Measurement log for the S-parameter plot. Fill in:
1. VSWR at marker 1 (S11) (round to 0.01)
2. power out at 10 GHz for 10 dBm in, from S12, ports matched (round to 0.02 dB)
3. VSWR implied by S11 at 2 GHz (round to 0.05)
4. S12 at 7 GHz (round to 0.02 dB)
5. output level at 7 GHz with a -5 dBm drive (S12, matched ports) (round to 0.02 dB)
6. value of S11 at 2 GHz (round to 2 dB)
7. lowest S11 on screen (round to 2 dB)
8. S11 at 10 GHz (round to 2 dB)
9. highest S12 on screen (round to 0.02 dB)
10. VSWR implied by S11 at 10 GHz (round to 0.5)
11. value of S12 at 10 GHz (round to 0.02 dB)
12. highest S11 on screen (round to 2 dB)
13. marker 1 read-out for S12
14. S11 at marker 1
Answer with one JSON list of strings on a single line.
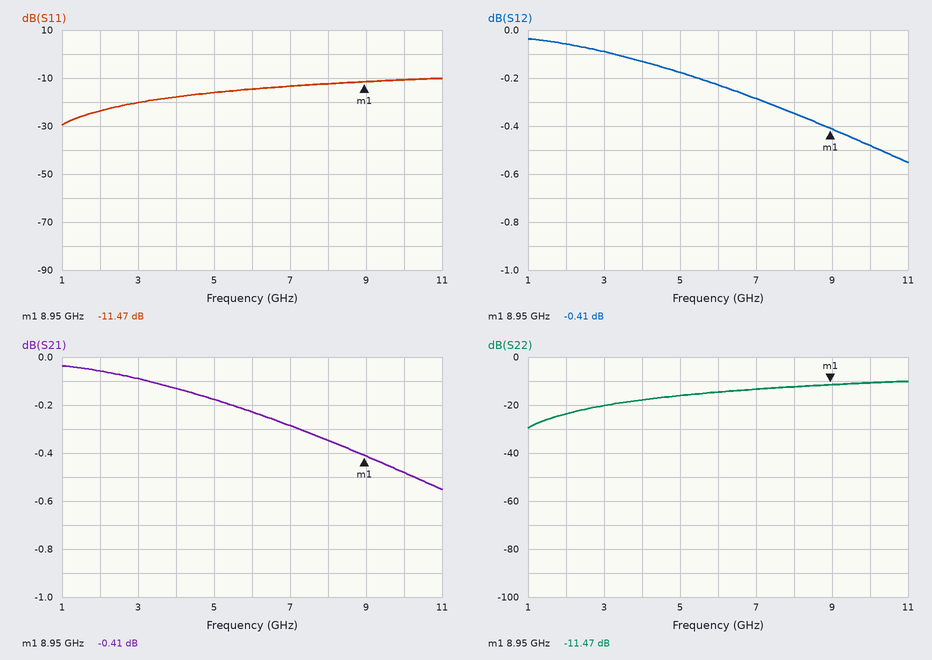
["1.73", "9.52 dBm", "1.15", "-0.28 dB", "-5.28 dBm", "-24 dB", "-30 dB", "-10 dB", "-0.04 dB", "2.0", "-0.48 dB", "-10 dB", "-0.41 dB", "-11.47 dB"]
